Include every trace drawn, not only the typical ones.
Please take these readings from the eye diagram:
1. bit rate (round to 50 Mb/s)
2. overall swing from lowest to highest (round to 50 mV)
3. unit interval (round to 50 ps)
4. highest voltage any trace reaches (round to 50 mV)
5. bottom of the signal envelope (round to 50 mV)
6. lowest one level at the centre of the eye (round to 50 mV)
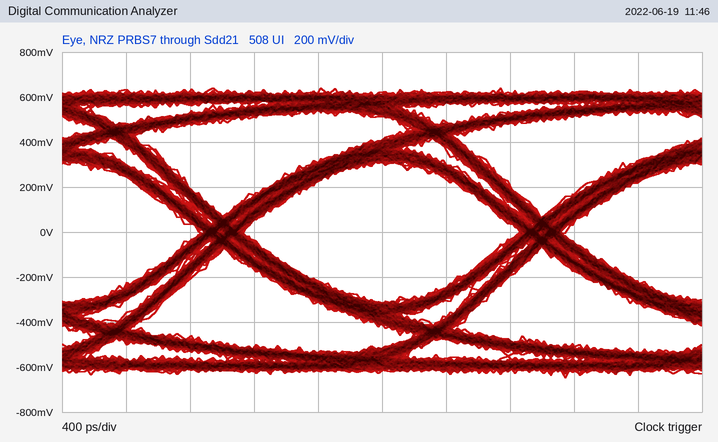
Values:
500 Mb/s
1.30 V
2.00 ns
650 mV
-650 mV
300 mV
